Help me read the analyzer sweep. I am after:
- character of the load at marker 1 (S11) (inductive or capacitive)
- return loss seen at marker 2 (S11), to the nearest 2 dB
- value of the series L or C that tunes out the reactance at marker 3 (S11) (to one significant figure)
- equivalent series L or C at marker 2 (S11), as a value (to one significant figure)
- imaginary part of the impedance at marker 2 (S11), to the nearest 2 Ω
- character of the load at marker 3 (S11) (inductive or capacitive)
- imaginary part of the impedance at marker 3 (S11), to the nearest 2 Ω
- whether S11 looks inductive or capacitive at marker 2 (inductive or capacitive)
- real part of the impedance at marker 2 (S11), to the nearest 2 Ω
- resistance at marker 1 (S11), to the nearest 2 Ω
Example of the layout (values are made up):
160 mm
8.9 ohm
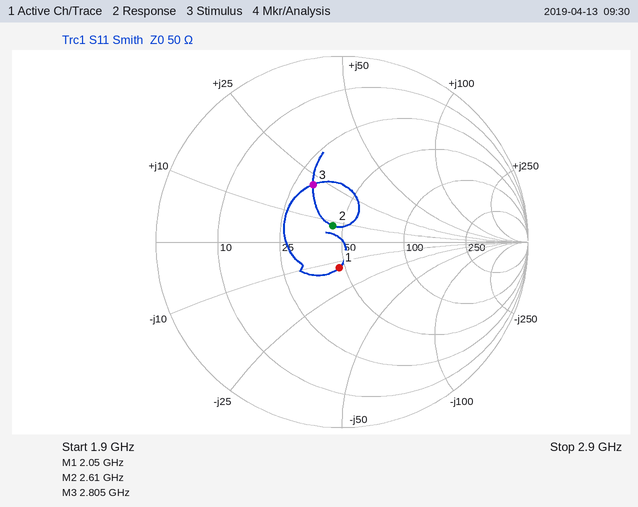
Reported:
capacitive
20 dB
3 pF
500 pH
+8 Ω
inductive
+22 Ω
inductive
44 Ω
46 Ω
